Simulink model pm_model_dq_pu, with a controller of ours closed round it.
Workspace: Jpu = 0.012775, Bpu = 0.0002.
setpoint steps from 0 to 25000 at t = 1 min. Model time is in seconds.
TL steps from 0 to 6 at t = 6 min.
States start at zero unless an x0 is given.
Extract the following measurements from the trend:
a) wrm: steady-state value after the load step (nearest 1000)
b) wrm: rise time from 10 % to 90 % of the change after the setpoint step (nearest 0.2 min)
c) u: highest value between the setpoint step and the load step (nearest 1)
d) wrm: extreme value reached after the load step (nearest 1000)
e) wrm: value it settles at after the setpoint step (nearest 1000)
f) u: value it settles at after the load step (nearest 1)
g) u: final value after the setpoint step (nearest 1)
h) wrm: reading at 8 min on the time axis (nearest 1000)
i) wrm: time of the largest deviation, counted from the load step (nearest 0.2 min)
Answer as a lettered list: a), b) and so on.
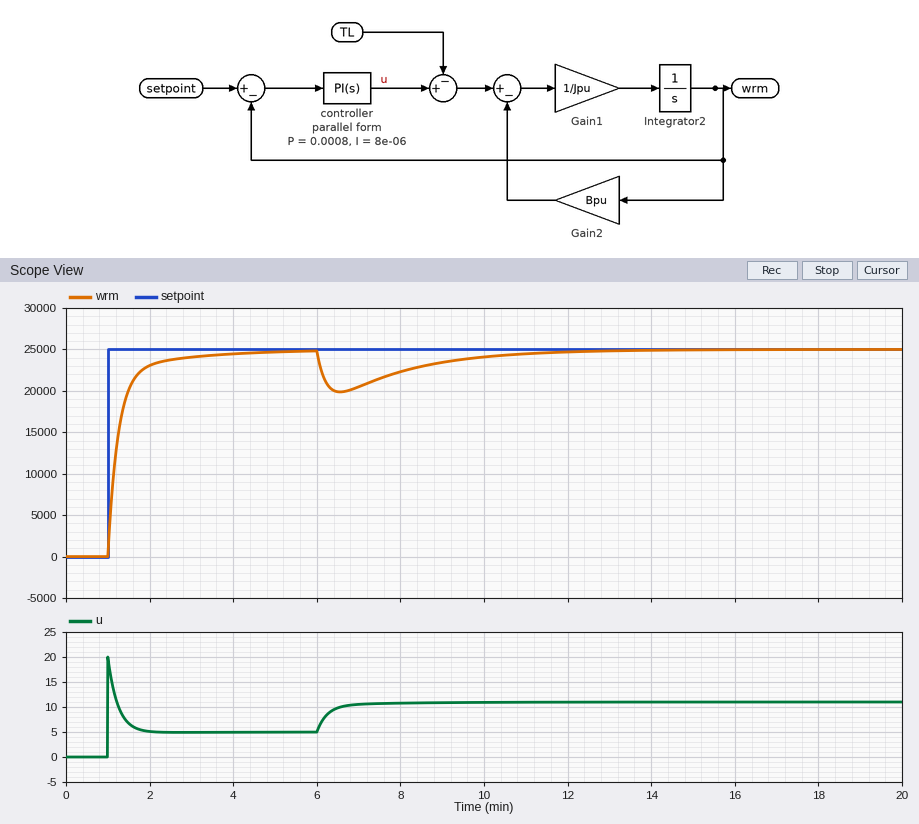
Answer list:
a) 25000
b) 0.8 min
c) 20
d) 20000
e) 25000
f) 11
g) 5
h) 22000
i) 0.6 min
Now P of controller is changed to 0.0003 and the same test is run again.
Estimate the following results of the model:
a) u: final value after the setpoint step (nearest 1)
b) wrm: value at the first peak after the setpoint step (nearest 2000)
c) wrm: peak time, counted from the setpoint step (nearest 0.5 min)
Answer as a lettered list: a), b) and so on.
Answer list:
a) 5
b) 26000
c) 2.0 min
